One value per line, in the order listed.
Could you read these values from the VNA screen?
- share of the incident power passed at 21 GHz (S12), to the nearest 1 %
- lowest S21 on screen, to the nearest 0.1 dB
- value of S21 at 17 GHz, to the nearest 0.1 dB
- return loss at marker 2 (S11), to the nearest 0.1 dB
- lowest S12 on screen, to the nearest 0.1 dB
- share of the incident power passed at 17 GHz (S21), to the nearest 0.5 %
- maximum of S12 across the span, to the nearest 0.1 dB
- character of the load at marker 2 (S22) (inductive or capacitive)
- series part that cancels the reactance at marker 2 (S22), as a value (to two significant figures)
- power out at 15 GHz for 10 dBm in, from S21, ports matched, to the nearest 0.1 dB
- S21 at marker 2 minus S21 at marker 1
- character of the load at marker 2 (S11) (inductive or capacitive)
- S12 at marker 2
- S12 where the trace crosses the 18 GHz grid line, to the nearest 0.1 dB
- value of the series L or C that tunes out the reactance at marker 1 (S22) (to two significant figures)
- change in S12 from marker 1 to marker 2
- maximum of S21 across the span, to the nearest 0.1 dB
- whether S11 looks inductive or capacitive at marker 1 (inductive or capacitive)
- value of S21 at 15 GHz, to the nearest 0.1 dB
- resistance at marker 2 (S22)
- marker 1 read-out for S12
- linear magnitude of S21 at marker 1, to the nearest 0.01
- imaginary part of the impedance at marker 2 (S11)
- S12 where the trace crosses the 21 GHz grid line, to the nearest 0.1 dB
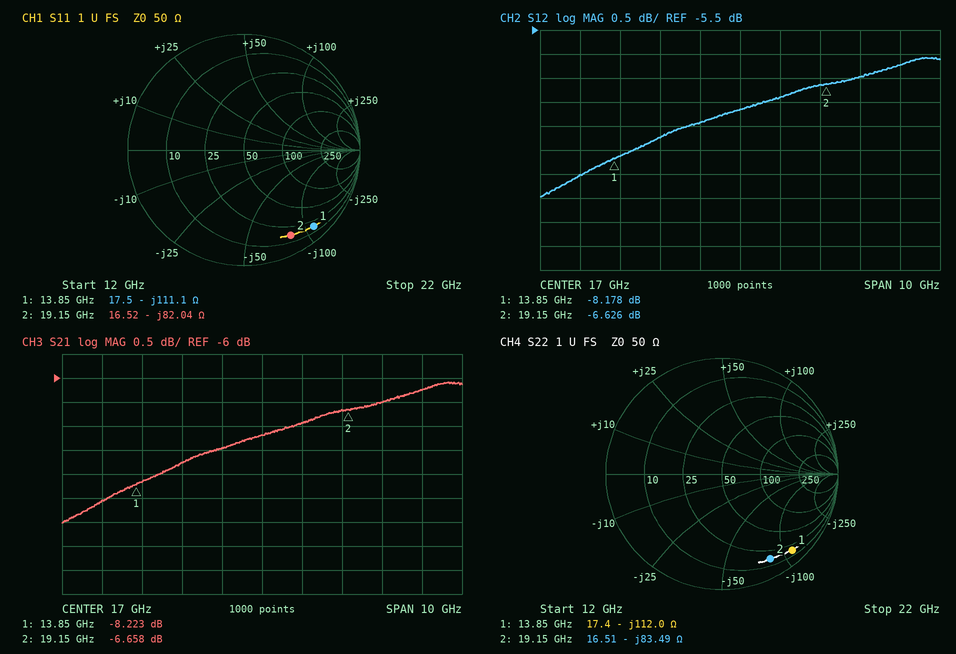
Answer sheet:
24 %
-9.0 dB
-7.2 dB
1.5 dB
-9.0 dB
19.0 %
-6.1 dB
capacitive
690 pH
2.2 dBm
1.565 dB
capacitive
-6.626 dB
-6.9 dB
1.3 nH
1.552 dB
-6.1 dB
capacitive
-7.8 dB
16.51 Ω
-8.178 dB
0.39
-82.04 Ω
-6.2 dB
